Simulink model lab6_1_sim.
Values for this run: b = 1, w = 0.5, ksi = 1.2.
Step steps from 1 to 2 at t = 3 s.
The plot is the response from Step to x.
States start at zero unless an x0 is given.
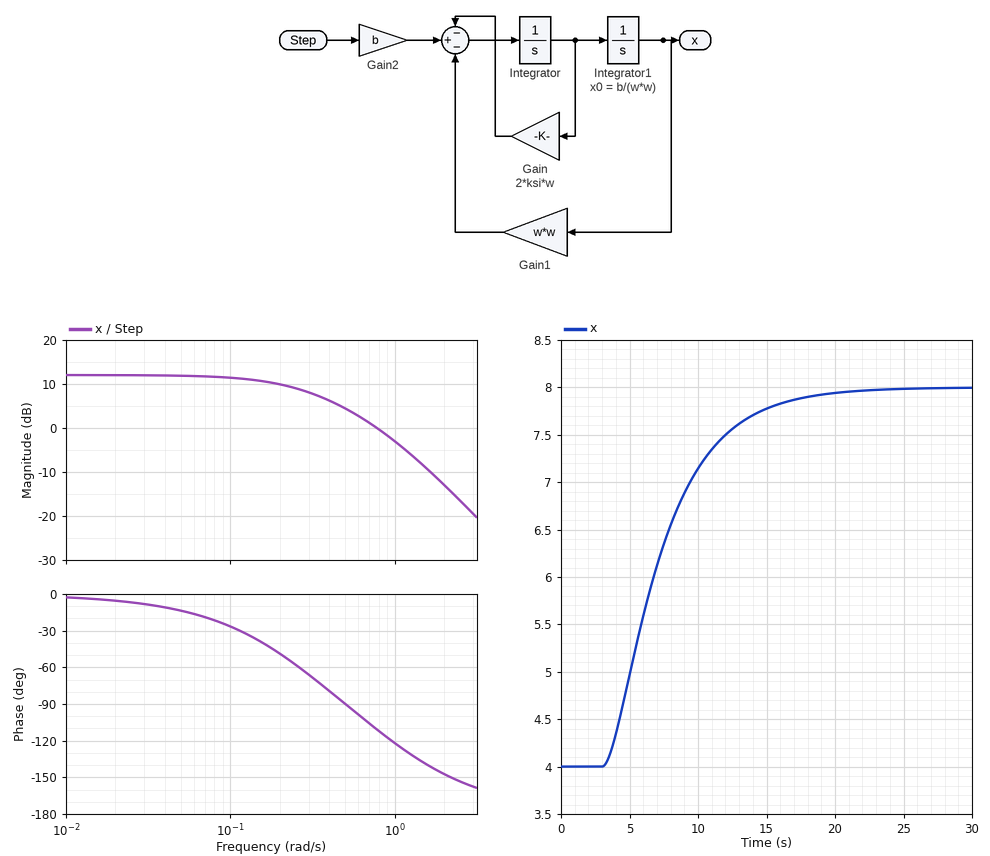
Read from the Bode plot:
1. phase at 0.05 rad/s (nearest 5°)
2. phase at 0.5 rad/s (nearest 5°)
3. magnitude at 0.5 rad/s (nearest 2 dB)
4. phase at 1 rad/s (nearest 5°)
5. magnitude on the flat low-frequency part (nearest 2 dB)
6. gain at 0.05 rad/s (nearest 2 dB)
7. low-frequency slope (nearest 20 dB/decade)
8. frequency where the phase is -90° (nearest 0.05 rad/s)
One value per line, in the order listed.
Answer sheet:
-15°
-90°
4 dB
-120°
12 dB
12 dB
0 dB/decade
0.50 rad/s
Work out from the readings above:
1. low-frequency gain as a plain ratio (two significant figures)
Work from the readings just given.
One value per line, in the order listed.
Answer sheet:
4.0
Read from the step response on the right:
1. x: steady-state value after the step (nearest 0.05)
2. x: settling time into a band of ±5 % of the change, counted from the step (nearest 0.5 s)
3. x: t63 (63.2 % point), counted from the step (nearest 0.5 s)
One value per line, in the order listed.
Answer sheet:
8.00
12.5 s
5.0 s
